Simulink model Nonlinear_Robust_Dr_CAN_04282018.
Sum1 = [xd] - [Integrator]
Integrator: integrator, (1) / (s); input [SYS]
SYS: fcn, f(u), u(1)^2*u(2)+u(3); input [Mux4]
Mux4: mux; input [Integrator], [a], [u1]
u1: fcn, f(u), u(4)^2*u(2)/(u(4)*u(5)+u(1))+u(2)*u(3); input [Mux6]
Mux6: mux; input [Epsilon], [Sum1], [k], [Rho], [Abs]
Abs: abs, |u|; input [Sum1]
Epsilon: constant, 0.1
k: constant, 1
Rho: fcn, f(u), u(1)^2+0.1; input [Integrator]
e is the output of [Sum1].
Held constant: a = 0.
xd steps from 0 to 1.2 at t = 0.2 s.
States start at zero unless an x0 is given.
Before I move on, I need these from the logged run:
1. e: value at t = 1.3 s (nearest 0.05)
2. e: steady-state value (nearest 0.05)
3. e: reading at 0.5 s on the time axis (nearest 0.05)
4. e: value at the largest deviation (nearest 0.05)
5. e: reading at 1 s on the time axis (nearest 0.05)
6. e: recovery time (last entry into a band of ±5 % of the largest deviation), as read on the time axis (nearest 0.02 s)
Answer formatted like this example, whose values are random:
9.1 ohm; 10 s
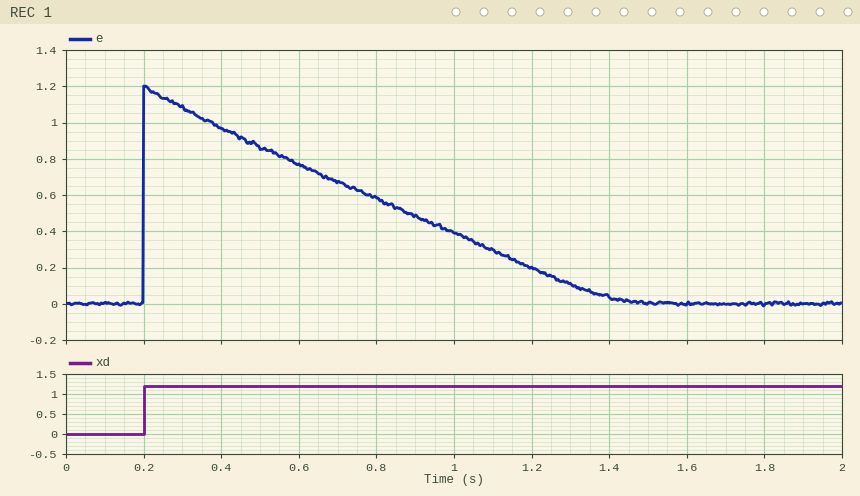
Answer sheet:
0.10; 0.00; 0.85; 1.20; 0.40; 1.36 s
